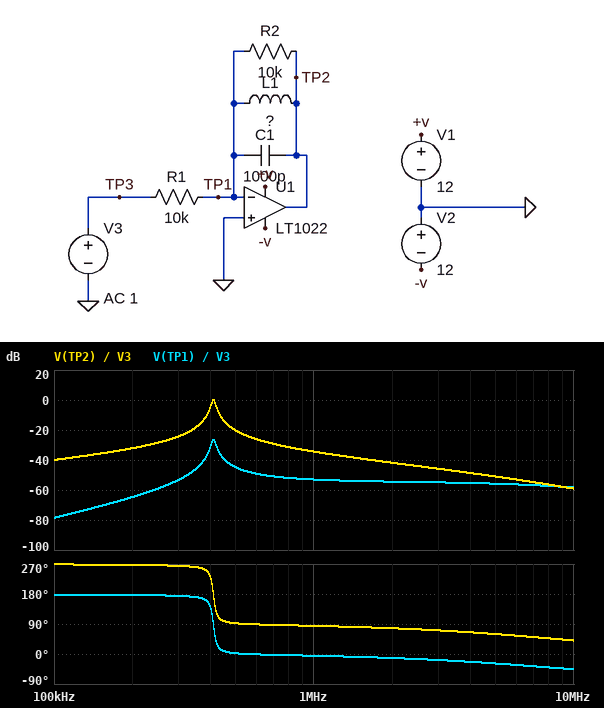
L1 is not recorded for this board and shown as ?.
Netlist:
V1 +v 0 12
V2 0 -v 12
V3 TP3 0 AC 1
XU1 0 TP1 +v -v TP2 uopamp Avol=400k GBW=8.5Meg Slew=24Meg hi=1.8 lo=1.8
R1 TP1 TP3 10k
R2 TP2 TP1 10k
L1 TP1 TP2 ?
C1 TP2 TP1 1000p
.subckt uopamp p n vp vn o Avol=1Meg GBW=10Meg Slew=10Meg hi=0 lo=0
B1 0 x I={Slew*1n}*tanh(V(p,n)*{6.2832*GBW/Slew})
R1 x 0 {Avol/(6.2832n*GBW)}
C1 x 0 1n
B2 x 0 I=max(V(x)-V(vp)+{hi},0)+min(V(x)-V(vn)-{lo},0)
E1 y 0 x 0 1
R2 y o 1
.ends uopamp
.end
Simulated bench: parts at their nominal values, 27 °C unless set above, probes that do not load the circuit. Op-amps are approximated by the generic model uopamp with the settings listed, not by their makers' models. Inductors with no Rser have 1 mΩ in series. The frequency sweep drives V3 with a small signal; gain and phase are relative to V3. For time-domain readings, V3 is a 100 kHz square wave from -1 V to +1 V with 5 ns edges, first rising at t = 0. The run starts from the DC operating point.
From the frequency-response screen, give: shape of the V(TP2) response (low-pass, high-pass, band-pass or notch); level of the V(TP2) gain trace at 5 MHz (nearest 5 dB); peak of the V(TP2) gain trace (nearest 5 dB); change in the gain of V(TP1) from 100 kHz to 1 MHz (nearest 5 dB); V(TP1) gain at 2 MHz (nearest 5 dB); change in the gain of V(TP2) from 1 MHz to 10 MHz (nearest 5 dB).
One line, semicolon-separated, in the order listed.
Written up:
band-pass; -50 dB; 0 dB; 25 dB; -55 dB; -25 dB
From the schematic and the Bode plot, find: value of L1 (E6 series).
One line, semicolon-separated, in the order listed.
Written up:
150 µH
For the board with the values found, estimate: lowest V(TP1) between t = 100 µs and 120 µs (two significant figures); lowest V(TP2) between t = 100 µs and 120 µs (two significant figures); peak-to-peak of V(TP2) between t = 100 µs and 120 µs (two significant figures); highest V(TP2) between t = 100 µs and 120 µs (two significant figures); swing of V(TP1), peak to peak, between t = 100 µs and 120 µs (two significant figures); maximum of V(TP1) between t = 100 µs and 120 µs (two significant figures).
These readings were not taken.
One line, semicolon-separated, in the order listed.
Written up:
-2.1 mV; -43 mV; 85 mV; 43 mV; 4.2 mV; 2.1 mV
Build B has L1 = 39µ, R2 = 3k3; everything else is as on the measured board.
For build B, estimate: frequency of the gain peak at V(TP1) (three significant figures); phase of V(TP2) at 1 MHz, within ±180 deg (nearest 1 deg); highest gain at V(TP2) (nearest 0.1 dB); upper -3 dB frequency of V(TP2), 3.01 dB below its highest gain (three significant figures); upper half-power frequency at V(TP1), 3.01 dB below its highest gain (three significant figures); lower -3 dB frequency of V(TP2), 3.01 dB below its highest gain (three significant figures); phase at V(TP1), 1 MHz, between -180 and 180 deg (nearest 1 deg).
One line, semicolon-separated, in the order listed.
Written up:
806 kHz; 91 deg; -9.7 dB; 830 kHz; 831 kHz; 781 kHz; 1 deg
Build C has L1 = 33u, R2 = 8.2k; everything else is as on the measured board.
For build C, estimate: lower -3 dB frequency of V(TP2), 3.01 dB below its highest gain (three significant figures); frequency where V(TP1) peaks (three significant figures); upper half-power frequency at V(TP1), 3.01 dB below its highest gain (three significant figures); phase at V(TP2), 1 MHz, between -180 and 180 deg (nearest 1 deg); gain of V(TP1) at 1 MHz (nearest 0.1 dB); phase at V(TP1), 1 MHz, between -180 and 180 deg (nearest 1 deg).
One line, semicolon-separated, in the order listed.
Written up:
866 kHz; 875 kHz; 885 kHz; 88 deg; -42.0 dB; -2 deg
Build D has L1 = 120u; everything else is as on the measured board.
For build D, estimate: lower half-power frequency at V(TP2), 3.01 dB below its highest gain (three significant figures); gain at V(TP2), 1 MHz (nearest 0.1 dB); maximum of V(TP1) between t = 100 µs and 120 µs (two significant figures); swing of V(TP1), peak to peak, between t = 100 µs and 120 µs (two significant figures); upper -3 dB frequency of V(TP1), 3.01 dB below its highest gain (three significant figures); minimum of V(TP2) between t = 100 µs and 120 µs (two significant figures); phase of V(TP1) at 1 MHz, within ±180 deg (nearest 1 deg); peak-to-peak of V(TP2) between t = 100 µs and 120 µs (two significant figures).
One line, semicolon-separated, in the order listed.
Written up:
451 kHz; -34.0 dB; 3.4 mV; 6.8 mV; 467 kHz; -61 mV; -5 deg; 120 mV
